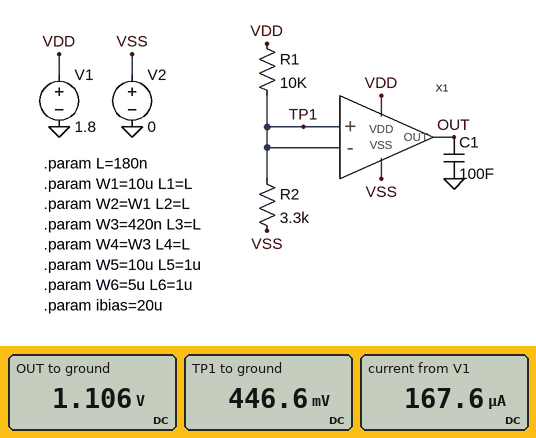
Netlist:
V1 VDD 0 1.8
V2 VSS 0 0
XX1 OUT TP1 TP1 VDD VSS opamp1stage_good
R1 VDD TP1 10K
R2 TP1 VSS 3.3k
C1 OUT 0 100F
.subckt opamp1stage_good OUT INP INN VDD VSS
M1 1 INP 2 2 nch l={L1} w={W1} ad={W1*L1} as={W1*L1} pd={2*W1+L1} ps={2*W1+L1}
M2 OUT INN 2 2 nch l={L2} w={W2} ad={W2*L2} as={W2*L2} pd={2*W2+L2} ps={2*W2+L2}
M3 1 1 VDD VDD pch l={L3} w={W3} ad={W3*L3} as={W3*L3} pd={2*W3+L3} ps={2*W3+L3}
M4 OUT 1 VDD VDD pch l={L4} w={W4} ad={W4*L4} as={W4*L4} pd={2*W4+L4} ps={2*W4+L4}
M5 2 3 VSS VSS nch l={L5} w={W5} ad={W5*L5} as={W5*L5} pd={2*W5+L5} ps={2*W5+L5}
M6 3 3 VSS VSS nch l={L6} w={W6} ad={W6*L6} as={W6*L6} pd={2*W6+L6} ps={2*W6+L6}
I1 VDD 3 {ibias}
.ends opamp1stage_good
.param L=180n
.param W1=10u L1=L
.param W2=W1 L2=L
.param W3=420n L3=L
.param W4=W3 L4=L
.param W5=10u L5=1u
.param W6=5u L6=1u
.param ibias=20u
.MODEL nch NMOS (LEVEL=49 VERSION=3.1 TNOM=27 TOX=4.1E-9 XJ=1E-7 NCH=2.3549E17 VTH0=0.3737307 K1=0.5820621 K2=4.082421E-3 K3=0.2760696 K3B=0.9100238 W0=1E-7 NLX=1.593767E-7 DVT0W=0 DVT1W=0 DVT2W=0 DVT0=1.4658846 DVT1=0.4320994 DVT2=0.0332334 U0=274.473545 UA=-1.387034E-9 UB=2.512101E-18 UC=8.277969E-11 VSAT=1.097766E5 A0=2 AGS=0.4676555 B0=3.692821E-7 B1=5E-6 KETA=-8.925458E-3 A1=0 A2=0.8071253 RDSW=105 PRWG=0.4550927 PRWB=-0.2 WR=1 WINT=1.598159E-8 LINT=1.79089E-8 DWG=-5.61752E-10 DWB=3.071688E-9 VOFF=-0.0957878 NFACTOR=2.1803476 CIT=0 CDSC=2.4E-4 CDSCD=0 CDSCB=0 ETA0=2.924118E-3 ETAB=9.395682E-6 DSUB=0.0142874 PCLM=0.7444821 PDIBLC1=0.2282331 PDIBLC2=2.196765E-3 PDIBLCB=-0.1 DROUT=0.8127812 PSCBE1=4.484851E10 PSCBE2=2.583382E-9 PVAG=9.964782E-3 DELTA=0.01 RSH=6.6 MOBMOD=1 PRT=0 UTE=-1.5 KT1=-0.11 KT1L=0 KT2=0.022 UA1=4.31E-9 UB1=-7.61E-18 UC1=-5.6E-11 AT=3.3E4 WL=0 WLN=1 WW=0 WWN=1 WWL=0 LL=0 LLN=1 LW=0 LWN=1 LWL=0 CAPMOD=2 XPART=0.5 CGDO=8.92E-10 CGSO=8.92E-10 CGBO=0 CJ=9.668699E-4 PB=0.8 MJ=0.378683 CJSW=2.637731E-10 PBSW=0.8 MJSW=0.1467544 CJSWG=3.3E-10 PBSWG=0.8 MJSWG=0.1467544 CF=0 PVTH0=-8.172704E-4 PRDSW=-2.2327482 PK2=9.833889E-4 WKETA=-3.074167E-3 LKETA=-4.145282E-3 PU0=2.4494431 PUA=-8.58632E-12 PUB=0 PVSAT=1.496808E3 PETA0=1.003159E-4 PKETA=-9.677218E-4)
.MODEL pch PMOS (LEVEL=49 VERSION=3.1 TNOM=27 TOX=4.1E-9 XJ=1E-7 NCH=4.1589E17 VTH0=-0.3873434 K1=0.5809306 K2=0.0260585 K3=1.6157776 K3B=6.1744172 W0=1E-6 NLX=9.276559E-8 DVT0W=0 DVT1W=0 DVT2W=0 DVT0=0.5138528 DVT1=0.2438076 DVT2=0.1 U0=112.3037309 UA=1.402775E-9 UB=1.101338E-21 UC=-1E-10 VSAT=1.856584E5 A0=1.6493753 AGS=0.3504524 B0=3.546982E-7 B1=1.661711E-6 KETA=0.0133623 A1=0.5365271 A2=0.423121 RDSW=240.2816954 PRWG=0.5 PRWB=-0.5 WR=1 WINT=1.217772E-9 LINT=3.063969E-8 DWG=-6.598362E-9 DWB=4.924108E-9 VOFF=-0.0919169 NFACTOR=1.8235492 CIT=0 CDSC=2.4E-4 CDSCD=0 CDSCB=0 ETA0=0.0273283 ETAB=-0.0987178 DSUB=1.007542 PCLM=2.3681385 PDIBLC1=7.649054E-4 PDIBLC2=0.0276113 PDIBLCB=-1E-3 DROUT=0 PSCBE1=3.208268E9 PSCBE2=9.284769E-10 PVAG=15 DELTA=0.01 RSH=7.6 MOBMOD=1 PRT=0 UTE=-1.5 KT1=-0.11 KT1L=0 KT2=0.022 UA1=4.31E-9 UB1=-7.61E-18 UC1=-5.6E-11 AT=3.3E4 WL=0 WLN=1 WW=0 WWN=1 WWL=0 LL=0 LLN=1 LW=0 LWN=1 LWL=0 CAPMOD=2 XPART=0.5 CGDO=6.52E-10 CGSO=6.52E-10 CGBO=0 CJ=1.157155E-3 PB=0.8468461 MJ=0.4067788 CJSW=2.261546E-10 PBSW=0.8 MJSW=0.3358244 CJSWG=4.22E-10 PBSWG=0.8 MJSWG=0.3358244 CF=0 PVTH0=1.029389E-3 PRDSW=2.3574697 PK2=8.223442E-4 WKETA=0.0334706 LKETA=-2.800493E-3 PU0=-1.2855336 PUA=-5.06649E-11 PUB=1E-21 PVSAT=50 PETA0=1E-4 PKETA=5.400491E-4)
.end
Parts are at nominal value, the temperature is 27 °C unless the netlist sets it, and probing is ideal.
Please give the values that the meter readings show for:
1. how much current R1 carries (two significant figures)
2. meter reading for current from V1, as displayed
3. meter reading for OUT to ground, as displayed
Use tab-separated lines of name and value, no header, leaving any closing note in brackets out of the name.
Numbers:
how much current R1 carries	140 µA
meter reading for current from V1, as displayed	167.6 µA
meter reading for OUT to ground, as displayed	1.106 V
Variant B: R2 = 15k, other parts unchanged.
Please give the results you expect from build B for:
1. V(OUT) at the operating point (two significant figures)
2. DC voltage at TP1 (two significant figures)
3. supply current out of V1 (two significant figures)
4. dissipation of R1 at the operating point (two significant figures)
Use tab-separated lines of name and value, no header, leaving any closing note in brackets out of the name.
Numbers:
V(OUT) at the operating point	890 mV
DC voltage at TP1	1.1 V
supply current out of V1	130 µA
dissipation of R1 at the operating point	52 µW
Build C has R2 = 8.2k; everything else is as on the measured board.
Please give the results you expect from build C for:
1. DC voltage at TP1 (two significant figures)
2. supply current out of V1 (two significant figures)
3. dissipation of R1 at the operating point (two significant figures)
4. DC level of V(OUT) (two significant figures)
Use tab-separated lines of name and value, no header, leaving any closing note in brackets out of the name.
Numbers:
DC voltage at TP1	810 mV
supply current out of V1	160 µA
dissipation of R1 at the operating point	98 µW
DC level of V(OUT)	900 mV
